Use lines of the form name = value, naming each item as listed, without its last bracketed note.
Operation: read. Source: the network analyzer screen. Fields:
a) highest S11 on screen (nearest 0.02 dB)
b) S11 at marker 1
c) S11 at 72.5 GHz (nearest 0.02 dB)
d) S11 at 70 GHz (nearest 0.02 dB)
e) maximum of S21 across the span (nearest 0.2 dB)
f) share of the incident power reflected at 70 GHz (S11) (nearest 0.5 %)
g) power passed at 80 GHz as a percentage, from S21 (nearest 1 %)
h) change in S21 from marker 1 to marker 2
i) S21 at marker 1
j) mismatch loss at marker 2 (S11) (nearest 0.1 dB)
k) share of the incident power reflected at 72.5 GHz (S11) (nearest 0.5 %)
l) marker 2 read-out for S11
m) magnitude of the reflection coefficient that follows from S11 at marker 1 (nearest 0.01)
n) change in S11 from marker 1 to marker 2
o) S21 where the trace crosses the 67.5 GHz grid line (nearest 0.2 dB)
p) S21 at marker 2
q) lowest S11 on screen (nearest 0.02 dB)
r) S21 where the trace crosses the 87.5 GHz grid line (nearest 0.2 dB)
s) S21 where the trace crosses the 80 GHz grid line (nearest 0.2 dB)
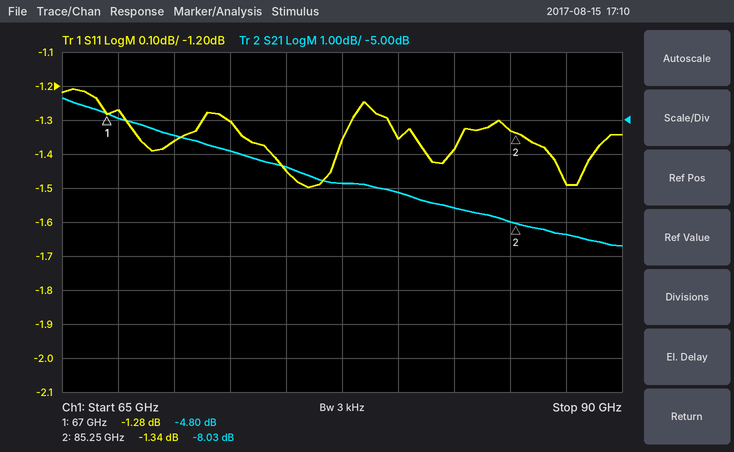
highest S11 on screen = -1.20 dB
S11 at marker 1 = -1.28 dB
S11 at 72.5 GHz = -1.30 dB
S11 at 70 GHz = -1.36 dB
maximum of S21 across the span = -4.4 dB
share of the incident power reflected at 70 GHz (S11) = 73.0 %
power passed at 80 GHz as a percentage, from S21 = 19 %
change in S21 from marker 1 to marker 2 = -3.23 dB
S21 at marker 1 = -4.80 dB
mismatch loss at marker 2 (S11) = 5.8 dB
share of the incident power reflected at 72.5 GHz (S11) = 74.0 %
marker 2 read-out for S11 = -1.34 dB
magnitude of the reflection coefficient that follows from S11 at marker 1 = 0.86
change in S11 from marker 1 to marker 2 = -0.06 dB
S21 where the trace crosses the 67.5 GHz grid line = -5.0 dB
S21 at marker 2 = -8.03 dB
lowest S11 on screen = -1.50 dB
S21 where the trace crosses the 87.5 GHz grid line = -8.4 dB
S21 where the trace crosses the 80 GHz grid line = -7.2 dB
